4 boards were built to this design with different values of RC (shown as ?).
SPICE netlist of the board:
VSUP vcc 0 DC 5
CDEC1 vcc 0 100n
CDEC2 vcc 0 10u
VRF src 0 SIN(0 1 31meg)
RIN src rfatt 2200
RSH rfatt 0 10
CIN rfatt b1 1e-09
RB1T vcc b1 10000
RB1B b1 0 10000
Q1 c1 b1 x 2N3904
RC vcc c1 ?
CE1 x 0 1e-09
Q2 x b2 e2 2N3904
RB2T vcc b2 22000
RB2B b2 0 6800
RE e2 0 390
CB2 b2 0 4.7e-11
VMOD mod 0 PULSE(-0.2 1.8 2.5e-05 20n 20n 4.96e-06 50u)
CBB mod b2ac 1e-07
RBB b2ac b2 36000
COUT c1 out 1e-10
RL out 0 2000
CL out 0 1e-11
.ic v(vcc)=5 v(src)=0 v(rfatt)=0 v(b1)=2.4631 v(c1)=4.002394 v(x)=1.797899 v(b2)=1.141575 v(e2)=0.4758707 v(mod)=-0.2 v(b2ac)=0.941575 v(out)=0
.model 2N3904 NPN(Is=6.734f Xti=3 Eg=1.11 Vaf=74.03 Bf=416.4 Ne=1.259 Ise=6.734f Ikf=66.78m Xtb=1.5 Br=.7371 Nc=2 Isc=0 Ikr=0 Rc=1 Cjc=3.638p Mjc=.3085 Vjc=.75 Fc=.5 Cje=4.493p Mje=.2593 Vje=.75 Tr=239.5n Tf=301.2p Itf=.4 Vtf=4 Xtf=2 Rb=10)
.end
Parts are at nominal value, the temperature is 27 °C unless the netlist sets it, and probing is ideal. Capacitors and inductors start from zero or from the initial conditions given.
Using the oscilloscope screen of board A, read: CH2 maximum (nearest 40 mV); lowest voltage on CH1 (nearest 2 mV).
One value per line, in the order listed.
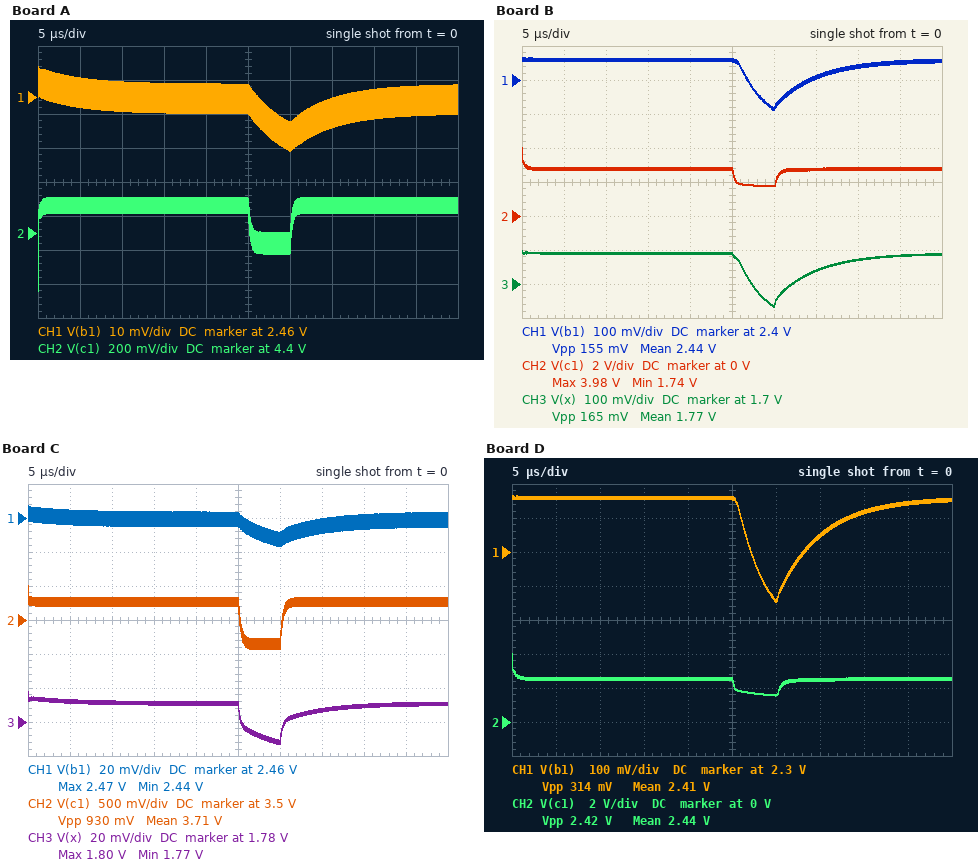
4.60 V
2.444 V
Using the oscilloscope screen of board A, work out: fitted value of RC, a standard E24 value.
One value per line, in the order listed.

390 Ω
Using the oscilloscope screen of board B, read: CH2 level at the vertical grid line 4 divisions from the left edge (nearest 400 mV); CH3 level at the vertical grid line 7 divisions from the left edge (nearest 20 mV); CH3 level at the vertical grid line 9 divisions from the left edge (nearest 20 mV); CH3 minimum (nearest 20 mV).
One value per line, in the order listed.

2.8 V
1.74 V
1.78 V
1.64 V
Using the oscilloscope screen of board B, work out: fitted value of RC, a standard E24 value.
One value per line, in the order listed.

2 kΩ
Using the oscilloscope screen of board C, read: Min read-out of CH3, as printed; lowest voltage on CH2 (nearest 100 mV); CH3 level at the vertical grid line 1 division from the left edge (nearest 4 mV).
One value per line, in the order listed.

1.77 V
3.1 V
1.792 V
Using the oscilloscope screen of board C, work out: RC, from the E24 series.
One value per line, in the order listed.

1.1 kΩ
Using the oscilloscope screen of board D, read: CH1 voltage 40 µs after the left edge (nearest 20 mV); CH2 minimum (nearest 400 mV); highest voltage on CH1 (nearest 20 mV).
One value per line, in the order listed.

2.42 V
1.6 V
2.46 V
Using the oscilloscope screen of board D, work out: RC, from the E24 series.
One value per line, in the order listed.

2.2 kΩ
